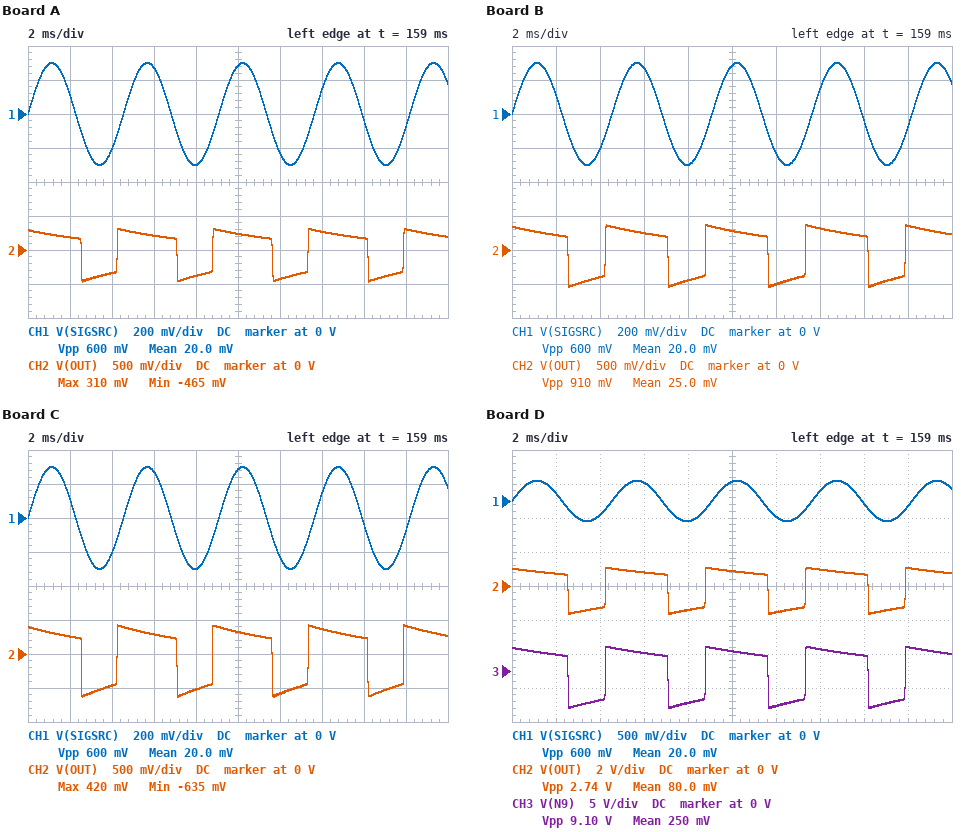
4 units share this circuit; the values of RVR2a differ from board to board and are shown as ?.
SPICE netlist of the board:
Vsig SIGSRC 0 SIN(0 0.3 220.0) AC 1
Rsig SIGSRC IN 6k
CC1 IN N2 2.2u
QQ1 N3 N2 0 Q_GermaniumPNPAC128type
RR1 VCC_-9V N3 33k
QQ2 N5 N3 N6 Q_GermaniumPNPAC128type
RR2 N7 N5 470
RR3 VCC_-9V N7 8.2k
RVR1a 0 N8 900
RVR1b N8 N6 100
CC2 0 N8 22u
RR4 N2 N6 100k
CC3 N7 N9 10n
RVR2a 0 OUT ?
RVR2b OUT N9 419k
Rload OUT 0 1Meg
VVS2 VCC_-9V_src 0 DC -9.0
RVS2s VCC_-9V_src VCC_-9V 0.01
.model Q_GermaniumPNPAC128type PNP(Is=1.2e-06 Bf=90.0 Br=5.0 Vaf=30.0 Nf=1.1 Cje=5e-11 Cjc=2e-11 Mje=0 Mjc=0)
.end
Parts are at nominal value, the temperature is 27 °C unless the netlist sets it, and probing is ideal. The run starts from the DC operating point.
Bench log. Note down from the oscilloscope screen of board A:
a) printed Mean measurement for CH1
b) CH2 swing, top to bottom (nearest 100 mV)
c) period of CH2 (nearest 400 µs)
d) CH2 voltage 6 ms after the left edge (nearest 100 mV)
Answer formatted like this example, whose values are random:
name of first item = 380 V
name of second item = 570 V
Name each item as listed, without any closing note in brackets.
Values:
printed Mean measurement for CH1 = 20.0 mV
CH2 swing, top to bottom = 800 mV
period of CH2 = 4.4 ms
CH2 voltage 6 ms after the left edge = 200 mV
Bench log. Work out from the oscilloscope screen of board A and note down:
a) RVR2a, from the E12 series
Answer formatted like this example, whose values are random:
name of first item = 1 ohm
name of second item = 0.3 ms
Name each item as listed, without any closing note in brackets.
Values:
RVR2a, from the E12 series = 39 kΩ
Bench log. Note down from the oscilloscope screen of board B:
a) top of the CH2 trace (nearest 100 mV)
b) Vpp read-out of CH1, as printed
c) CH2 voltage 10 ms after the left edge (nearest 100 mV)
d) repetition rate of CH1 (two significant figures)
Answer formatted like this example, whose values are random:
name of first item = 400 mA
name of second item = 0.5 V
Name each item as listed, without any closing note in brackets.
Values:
top of the CH2 trace = 400 mV
Vpp read-out of CH1, as printed = 600 mV
CH2 voltage 10 ms after the left edge = 300 mV
repetition rate of CH1 = 220 Hz
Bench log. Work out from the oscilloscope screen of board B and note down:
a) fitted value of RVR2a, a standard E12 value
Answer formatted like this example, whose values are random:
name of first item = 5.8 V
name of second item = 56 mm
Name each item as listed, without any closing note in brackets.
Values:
fitted value of RVR2a, a standard E12 value = 47 kΩ
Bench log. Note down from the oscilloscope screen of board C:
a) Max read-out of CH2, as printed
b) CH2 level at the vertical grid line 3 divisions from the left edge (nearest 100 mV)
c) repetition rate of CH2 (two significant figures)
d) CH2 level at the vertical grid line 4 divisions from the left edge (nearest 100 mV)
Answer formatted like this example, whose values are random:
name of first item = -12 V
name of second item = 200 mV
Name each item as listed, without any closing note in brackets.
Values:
Max read-out of CH2, as printed = 420 mV
CH2 level at the vertical grid line 3 divisions from the left edge = 300 mV
repetition rate of CH2 = 220 Hz
CH2 level at the vertical grid line 4 divisions from the left edge = -500 mV
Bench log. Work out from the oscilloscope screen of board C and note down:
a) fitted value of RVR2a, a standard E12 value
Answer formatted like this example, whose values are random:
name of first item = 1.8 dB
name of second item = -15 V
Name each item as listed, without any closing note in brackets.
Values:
fitted value of RVR2a, a standard E12 value = 56 kΩ
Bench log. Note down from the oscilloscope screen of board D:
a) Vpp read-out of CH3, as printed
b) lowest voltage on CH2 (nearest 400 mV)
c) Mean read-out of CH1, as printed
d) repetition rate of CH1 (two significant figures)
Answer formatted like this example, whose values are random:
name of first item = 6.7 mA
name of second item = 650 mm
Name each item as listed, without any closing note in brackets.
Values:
Vpp read-out of CH3, as printed = 9.10 V
lowest voltage on CH2 = -1.6 V
Mean read-out of CH1, as printed = 20.0 mV
repetition rate of CH1 = 220 Hz
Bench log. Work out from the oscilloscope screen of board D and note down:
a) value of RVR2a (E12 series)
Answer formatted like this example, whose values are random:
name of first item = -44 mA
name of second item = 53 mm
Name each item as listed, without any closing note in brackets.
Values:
value of RVR2a = 220 kΩ
